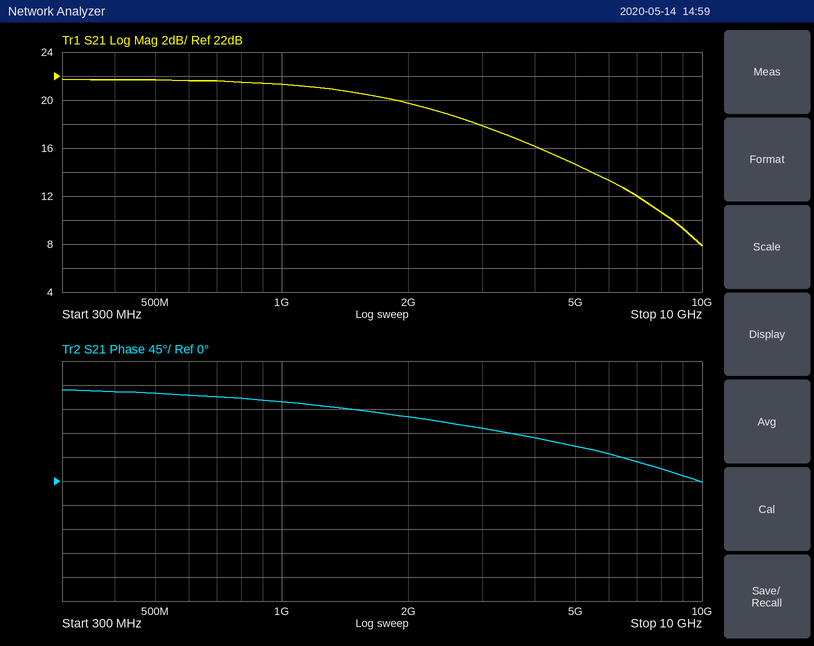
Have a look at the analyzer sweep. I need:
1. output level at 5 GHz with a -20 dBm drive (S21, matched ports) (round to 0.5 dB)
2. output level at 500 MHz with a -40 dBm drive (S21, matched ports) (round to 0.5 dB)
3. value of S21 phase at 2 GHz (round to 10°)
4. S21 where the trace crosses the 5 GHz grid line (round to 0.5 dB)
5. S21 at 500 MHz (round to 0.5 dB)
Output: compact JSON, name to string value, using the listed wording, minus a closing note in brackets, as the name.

{"output level at 5 GHz with a -20 dBm drive (S21, matched ports)": "-5.5 dBm", "output level at 500 MHz with a -40 dBm drive (S21, matched ports)": "-18.5 dBm", "value of S21 phase at 2 GHz": "120°", "S21 where the trace crosses the 5 GHz grid line": "14.5 dB", "S21 at 500 MHz": "21.5 dB"}
